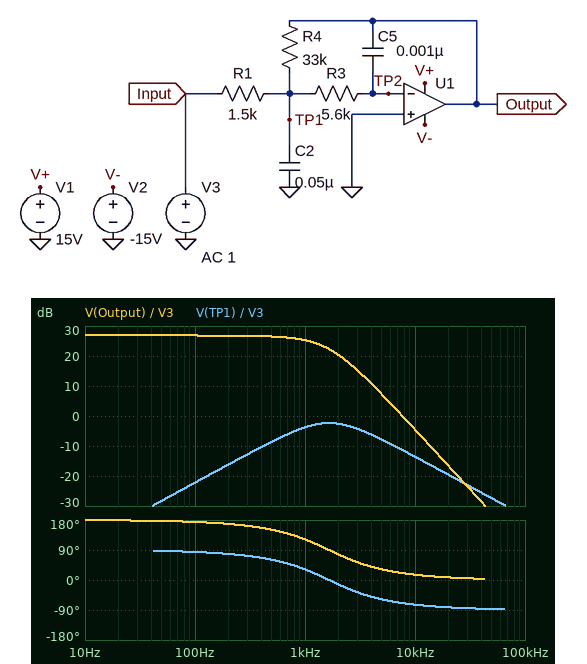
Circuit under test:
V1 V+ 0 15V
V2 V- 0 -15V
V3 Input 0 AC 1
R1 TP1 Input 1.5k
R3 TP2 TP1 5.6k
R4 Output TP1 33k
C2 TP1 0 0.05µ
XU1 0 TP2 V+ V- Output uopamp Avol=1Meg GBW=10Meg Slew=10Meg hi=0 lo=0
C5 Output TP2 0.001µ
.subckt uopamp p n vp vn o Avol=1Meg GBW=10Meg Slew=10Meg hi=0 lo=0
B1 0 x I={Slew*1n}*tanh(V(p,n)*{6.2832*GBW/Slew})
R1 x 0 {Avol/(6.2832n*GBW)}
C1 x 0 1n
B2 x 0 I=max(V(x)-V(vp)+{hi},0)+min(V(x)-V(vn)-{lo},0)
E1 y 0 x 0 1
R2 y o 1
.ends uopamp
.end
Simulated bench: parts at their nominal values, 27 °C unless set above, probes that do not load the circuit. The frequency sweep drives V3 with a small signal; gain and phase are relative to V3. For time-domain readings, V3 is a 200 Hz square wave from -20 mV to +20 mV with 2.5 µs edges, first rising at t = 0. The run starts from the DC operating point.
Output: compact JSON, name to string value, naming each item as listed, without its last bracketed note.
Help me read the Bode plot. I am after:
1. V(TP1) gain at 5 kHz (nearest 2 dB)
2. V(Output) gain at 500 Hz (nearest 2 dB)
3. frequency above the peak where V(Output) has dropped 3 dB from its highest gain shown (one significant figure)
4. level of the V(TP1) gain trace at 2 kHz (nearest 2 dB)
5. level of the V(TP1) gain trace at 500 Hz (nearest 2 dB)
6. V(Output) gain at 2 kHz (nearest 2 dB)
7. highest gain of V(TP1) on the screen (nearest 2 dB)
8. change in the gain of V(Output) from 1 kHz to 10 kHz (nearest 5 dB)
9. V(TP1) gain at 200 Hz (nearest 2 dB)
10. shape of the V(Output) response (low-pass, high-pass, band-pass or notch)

{"V(TP1) gain at 5 kHz": "-8 dB", "V(Output) gain at 500 Hz": "26 dB", "frequency above the peak where V(Output) has dropped 3 dB from its highest gain shown": "1 kHz", "level of the V(TP1) gain trace at 2 kHz": "-2 dB", "level of the V(TP1) gain trace at 500 Hz": "-8 dB", "V(Output) gain at 2 kHz": "20 dB", "highest gain of V(TP1) on the screen": "-2 dB", "change in the gain of V(Output) from 1 kHz to 10 kHz": "-30 dB", "V(TP1) gain at 200 Hz": "-16 dB", "shape of the V(Output) response": "low-pass"}
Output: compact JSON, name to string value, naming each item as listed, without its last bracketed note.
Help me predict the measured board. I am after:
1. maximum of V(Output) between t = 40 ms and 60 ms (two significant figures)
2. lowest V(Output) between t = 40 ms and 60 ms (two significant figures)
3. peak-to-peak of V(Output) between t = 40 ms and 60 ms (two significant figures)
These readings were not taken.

{"maximum of V(Output) between t = 40 ms and 60 ms": "450 mV", "lowest V(Output) between t = 40 ms and 60 ms": "-450 mV", "peak-to-peak of V(Output) between t = 40 ms and 60 ms": "890 mV"}
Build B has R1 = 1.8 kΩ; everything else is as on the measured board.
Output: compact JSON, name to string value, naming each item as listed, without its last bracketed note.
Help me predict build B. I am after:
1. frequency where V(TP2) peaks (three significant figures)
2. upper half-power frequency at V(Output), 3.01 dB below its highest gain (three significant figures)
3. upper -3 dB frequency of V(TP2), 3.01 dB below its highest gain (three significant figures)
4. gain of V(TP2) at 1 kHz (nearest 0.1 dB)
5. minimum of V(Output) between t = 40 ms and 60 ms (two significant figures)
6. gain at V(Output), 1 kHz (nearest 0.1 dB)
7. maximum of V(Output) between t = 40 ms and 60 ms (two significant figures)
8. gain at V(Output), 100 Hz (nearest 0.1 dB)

{"frequency where V(TP2) peaks": "1.65 kHz", "upper half-power frequency at V(Output), 3.01 dB below its highest gain": "1.59 kHz", "upper -3 dB frequency of V(TP2), 3.01 dB below its highest gain": "3.27 kHz", "gain of V(TP2) at 1 kHz": "-55.5 dB", "minimum of V(Output) between t = 40 ms and 60 ms": "-390 mV", "gain at V(Output), 1 kHz": "24.5 dB", "maximum of V(Output) between t = 40 ms and 60 ms": "390 mV", "gain at V(Output), 100 Hz": "25.3 dB"}
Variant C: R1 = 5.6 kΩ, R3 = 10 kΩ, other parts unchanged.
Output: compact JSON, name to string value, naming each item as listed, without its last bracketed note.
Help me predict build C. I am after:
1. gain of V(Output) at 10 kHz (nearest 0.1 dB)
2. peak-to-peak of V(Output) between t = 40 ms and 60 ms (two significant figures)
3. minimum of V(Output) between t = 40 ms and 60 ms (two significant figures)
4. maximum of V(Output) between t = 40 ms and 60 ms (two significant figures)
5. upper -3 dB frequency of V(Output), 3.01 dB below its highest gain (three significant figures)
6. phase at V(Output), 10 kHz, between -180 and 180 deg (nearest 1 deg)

{"gain of V(Output) at 10 kHz": "-20.8 dB", "peak-to-peak of V(Output) between t = 40 ms and 60 ms": "360 mV", "minimum of V(Output) between t = 40 ms and 60 ms": "-180 mV", "maximum of V(Output) between t = 40 ms and 60 ms": "180 mV", "upper -3 dB frequency of V(Output), 3.01 dB below its highest gain": "1.47 kHz", "phase at V(Output), 10 kHz, between -180 and 180 deg": "6 deg"}
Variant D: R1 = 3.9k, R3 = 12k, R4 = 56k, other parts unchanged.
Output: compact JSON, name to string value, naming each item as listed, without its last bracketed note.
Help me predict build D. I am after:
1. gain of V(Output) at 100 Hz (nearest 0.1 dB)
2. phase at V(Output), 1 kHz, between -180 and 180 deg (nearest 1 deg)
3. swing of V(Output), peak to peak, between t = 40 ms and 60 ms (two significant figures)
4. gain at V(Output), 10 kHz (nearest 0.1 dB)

{"gain of V(Output) at 100 Hz": "23.2 dB", "phase at V(Output), 1 kHz, between -180 and 180 deg": "78 deg", "swing of V(Output), peak to peak, between t = 40 ms and 60 ms": "650 mV", "gain at V(Output), 10 kHz": "-19.3 dB"}
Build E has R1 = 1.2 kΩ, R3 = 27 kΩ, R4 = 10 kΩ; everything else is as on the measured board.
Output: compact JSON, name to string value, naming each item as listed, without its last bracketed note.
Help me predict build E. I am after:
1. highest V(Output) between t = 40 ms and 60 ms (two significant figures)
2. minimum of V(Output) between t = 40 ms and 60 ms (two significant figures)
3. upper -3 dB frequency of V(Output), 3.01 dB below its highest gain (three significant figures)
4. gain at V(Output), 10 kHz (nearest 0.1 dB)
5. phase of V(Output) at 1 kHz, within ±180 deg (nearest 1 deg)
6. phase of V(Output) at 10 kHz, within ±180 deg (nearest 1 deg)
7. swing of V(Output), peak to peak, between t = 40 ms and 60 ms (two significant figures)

{"highest V(Output) between t = 40 ms and 60 ms": "170 mV", "minimum of V(Output) between t = 40 ms and 60 ms": "-170 mV", "upper -3 dB frequency of V(Output), 3.01 dB below its highest gain": "745 Hz", "gain at V(Output), 10 kHz": "-16.4 dB", "phase of V(Output) at 1 kHz, within ±180 deg": "106 deg", "phase of V(Output) at 10 kHz, within ±180 deg": "17 deg", "swing of V(Output), peak to peak, between t = 40 ms and 60 ms": "330 mV"}
